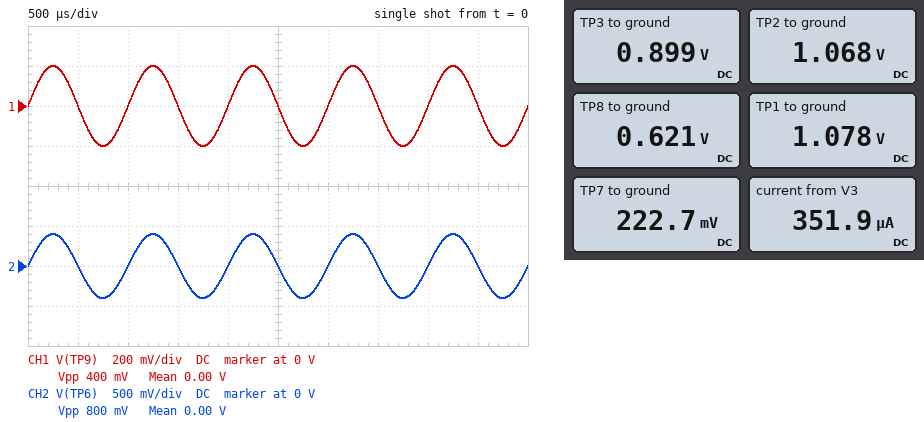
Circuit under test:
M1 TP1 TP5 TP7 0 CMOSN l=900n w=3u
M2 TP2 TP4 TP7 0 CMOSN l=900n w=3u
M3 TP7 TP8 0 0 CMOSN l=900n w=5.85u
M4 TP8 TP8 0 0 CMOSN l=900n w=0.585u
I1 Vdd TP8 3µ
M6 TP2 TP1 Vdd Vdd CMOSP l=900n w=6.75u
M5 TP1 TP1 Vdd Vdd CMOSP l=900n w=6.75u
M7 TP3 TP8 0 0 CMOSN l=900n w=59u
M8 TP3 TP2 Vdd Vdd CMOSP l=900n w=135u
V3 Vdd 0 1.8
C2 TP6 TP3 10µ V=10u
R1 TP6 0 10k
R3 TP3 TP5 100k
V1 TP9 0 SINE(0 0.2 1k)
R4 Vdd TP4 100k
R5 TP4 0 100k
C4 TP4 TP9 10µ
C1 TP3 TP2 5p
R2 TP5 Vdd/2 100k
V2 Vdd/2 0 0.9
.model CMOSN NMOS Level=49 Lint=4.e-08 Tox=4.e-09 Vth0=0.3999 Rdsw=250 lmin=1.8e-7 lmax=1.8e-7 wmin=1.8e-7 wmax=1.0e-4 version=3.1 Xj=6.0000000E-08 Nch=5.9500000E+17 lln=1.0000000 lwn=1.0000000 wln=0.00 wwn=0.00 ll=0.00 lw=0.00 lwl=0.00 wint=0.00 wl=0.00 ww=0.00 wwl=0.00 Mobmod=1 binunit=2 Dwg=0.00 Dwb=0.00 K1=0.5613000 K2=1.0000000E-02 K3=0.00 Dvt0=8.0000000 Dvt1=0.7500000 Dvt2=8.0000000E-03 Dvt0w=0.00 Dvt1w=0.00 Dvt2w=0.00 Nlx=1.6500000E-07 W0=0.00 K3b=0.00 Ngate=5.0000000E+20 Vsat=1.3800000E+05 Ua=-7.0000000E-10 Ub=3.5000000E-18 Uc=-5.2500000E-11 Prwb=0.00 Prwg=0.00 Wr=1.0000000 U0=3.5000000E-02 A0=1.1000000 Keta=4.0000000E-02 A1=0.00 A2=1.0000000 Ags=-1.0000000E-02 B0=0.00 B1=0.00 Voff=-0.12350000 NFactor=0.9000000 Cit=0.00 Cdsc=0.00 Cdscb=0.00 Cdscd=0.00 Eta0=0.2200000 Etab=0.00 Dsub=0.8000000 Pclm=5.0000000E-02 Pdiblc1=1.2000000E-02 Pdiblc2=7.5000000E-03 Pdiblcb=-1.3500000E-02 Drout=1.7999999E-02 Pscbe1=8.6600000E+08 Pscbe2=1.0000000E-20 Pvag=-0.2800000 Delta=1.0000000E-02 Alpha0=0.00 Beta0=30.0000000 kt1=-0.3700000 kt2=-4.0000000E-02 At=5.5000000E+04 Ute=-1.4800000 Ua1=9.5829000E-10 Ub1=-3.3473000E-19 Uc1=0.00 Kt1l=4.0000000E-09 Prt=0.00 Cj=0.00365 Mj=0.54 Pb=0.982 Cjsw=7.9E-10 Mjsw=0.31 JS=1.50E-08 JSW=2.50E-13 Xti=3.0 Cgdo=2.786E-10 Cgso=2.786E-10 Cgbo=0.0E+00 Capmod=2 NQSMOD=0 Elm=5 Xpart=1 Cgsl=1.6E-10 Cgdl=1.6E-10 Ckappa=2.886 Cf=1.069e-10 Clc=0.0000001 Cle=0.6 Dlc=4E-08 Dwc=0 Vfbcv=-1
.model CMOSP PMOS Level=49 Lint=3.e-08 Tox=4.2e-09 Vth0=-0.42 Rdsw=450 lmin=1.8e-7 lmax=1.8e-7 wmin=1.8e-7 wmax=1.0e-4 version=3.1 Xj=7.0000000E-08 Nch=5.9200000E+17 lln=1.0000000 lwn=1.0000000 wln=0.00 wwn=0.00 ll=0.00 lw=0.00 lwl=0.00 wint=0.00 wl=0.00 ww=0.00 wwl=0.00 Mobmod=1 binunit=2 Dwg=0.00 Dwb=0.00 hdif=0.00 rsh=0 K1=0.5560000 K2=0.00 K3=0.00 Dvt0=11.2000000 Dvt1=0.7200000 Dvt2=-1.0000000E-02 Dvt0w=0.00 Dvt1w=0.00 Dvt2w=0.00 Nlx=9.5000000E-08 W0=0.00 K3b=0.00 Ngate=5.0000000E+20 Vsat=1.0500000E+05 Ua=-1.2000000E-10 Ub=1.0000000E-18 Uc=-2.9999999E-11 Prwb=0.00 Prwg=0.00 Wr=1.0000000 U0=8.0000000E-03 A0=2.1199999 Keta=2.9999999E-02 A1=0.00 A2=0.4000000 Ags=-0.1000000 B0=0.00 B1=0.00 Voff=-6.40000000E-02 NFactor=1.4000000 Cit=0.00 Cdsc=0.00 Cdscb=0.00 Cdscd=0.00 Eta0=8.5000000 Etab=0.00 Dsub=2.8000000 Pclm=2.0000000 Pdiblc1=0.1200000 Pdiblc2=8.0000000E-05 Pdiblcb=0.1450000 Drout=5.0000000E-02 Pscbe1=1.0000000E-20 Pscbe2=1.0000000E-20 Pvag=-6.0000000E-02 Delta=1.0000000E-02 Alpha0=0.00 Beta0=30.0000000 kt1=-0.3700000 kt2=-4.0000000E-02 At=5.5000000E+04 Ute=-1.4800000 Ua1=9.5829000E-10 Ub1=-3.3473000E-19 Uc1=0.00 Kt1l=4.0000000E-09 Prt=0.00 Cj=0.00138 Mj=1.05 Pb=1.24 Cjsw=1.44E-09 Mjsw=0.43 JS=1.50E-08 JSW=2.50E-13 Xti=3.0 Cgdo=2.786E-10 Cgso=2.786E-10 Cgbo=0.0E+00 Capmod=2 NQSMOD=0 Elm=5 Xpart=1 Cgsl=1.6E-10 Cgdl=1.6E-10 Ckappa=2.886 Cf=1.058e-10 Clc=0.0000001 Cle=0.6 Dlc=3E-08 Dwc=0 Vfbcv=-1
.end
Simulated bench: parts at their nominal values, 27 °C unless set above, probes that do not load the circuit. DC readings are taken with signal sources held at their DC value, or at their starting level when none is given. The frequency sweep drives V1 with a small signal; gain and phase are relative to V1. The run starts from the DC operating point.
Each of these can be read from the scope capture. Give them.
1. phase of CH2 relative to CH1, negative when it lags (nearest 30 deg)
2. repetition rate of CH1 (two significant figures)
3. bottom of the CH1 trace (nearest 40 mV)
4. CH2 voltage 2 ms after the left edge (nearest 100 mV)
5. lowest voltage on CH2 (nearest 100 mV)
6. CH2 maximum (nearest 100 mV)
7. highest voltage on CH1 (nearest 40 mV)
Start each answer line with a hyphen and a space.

- 0 deg
- 1.0 kHz
- -200 mV
- 0 V
- -400 mV
- 400 mV
- 200 mV
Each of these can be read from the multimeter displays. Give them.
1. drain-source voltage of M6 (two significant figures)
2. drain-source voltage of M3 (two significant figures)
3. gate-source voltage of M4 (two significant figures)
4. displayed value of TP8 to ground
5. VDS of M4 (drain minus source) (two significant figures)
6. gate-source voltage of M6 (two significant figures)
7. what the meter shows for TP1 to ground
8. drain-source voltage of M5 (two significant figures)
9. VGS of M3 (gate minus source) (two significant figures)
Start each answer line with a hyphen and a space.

- -730 mV
- 220 mV
- 620 mV
- 0.621 V
- 620 mV
- -720 mV
- 1.078 V
- -720 mV
- 620 mV
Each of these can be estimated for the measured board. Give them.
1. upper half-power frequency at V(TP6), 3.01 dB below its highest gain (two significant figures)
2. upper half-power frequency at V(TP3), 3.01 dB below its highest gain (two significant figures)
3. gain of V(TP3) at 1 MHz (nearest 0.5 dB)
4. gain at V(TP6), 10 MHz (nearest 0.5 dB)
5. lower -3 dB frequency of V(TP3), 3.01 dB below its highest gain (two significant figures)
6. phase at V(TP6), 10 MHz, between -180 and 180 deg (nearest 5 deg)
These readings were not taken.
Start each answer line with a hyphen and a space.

- 2.1 MHz
- 2.1 MHz
- 5.0 dB
- -8.5 dB
- 320 mHz
- -95 deg
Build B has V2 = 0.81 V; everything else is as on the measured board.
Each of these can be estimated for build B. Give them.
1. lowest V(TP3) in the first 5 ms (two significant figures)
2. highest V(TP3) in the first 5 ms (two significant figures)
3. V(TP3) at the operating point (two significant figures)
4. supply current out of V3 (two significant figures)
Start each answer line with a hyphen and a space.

- 590 mV
- 1.4 V
- 990 mV
- 360 µA
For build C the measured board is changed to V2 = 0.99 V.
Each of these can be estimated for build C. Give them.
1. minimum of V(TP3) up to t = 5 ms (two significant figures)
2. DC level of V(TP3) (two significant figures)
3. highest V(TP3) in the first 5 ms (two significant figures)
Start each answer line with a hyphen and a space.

- 410 mV
- 810 mV
- 1.2 V
